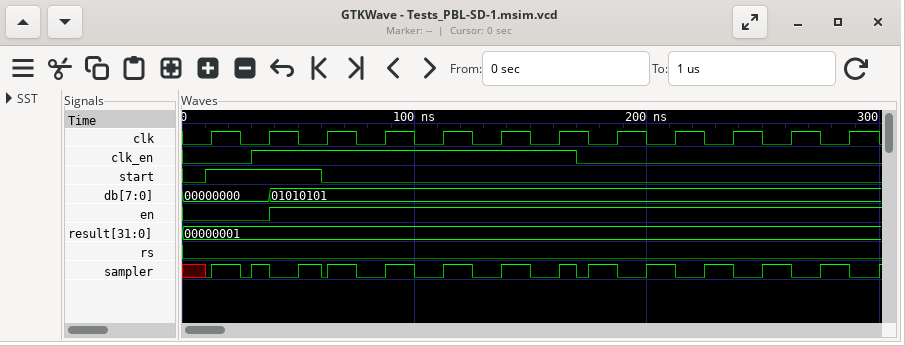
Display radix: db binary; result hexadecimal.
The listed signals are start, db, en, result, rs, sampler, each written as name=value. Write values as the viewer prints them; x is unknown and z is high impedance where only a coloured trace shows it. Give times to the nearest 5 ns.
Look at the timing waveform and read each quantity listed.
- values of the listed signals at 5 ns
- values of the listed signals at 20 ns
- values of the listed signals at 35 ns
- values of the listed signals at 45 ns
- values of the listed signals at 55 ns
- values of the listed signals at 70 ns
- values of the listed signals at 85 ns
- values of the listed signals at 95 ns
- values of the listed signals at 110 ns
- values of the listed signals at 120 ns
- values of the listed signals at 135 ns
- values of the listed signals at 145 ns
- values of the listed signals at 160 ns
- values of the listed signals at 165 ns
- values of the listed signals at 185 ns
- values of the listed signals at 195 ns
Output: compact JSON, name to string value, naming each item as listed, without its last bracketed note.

{"values of the listed signals at 5 ns": "start=0, db=00000000, en=0, result=00000001, rs=0, sampler=x", "values of the listed signals at 20 ns": "start=1, db=00000000, en=0, result=00000001, rs=0, sampler=1", "values of the listed signals at 35 ns": "start=1, db=00000000, en=0, result=00000001, rs=0, sampler=1", "values of the listed signals at 45 ns": "start=1, db=01010101, en=1, result=00000001, rs=0, sampler=0", "values of the listed signals at 55 ns": "start=1, db=01010101, en=1, result=00000001, rs=0, sampler=1", "values of the listed signals at 70 ns": "start=0, db=01010101, en=1, result=00000001, rs=0, sampler=1", "values of the listed signals at 85 ns": "start=0, db=01010101, en=1, result=00000001, rs=0, sampler=0", "values of the listed signals at 95 ns": "start=0, db=01010101, en=1, result=00000001, rs=0, sampler=1", "values of the listed signals at 110 ns": "start=0, db=01010101, en=1, result=00000001, rs=0, sampler=0", "values of the listed signals at 120 ns": "start=0, db=01010101, en=1, result=00000001, rs=0, sampler=1", "values of the listed signals at 135 ns": "start=0, db=01010101, en=1, result=00000001, rs=0, sampler=0", "values of the listed signals at 145 ns": "start=0, db=01010101, en=1, result=00000001, rs=0, sampler=1", "values of the listed signals at 160 ns": "start=0, db=01010101, en=1, result=00000001, rs=0, sampler=0", "values of the listed signals at 165 ns": "start=0, db=01010101, en=1, result=00000001, rs=0, sampler=1", "values of the listed signals at 185 ns": "start=0, db=01010101, en=1, result=00000001, rs=0, sampler=1", "values of the listed signals at 195 ns": "start=0, db=01010101, en=1, result=00000001, rs=0, sampler=0"}
